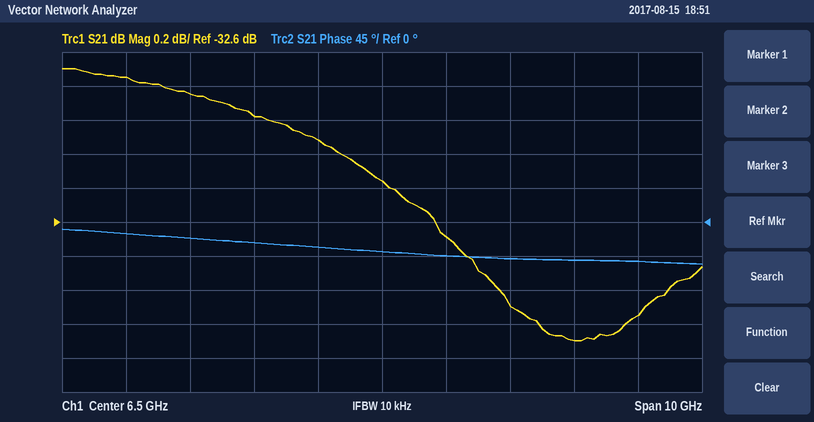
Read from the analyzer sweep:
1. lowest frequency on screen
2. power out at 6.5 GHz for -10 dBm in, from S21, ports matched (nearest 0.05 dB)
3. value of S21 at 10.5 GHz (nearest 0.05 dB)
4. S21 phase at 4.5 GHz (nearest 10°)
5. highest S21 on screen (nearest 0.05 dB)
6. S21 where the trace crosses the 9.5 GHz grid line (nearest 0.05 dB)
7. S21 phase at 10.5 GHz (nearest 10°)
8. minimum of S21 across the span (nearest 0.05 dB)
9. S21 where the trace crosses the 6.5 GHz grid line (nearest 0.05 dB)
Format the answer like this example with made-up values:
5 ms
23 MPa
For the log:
1.5 GHz
-42.35 dBm
-33.15 dB
-30°
-31.70 dB
-33.30 dB
-50°
-33.30 dB
-32.35 dB
